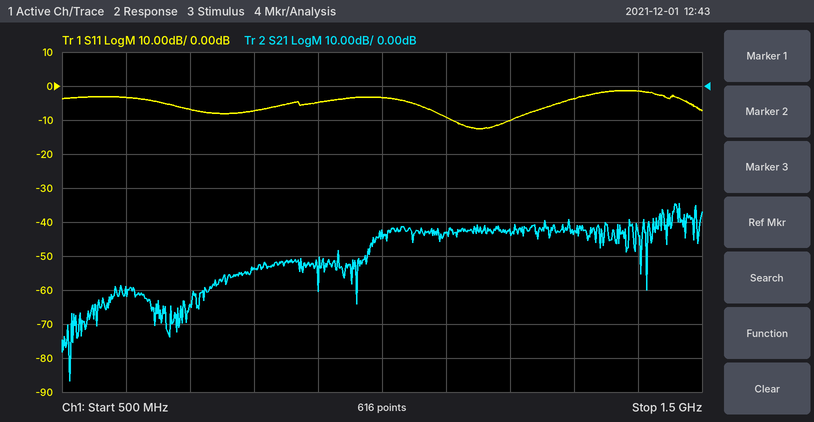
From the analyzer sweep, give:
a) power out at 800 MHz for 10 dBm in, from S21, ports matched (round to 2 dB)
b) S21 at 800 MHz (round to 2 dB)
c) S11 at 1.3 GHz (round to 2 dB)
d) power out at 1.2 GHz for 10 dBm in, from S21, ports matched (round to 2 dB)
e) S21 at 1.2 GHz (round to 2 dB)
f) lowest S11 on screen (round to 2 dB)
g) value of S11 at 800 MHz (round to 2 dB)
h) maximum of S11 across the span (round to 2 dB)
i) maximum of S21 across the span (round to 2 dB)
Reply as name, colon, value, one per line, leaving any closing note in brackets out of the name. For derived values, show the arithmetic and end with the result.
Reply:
power out at 800 MHz for 10 dBm in, from S21, ports matched: 10 dBm + (-54 dB) = -44 dBm
S21 at 800 MHz: -54 dB
S11 at 1.3 GHz: -4 dB
power out at 1.2 GHz for 10 dBm in, from S21, ports matched: 10 dBm + (-42 dB) = -32 dBm
S21 at 1.2 GHz: -42 dB
lowest S11 on screen: -12 dB
value of S11 at 800 MHz: -8 dB
maximum of S11 across the span: -2 dB
maximum of S21 across the span: -34 dB
